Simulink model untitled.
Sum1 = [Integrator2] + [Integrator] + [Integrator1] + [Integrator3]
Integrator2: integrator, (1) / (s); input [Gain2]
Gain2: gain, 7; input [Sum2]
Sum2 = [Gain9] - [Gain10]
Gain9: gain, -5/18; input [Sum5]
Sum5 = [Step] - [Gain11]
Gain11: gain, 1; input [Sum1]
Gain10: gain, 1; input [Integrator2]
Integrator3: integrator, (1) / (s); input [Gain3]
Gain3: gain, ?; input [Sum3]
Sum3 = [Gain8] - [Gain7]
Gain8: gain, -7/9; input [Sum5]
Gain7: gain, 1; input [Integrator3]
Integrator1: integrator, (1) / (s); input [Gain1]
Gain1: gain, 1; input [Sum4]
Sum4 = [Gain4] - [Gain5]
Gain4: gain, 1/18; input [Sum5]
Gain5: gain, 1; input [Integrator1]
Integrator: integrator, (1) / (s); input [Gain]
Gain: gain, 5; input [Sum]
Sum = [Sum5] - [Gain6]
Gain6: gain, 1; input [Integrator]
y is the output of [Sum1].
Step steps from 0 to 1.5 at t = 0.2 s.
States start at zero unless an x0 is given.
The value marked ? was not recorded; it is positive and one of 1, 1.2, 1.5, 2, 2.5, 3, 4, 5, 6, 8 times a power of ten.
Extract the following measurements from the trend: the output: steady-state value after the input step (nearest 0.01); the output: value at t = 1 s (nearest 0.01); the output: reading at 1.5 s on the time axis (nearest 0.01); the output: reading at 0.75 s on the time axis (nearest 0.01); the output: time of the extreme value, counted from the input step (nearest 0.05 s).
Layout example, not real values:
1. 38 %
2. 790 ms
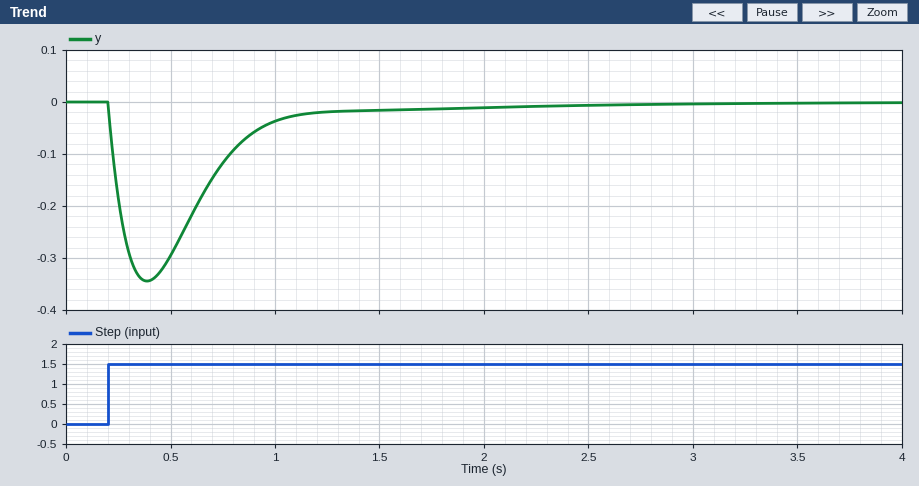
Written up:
1. 0.00
2. -0.04
3. -0.02
4. -0.12
5. 0.20 s
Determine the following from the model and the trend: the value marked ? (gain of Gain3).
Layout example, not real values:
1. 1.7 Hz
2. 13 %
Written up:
1. 8
